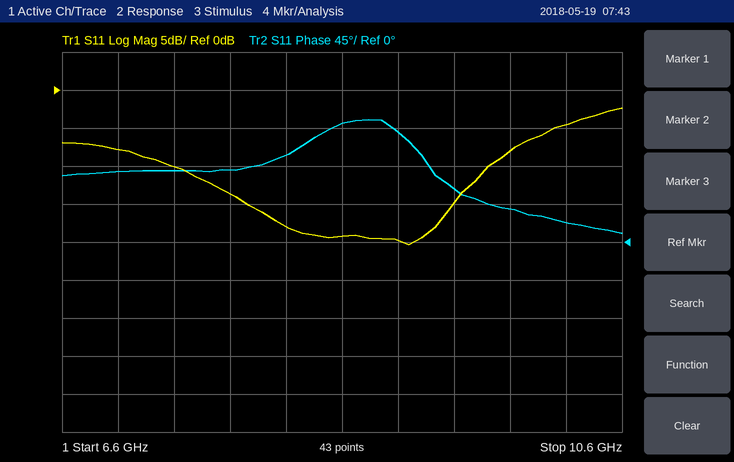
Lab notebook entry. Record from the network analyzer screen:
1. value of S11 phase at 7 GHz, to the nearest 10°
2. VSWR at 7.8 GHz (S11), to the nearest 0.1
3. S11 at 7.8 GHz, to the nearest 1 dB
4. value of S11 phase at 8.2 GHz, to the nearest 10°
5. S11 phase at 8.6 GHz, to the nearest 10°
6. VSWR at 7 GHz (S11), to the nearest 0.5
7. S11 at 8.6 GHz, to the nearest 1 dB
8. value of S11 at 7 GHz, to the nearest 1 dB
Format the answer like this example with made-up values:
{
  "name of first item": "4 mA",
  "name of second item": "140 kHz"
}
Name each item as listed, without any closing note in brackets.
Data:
{
  "value of S11 phase at 7 GHz, to the nearest 10°": "80°",
  "VSWR at 7.8 GHz (S11), to the nearest 0.1": "1.5",
  "S11 at 7.8 GHz, to the nearest 1 dB": "-14 dB",
  "value of S11 phase at 8.2 GHz, to the nearest 10°": "100°",
  "S11 phase at 8.6 GHz, to the nearest 10°": "140°",
  "VSWR at 7 GHz (S11), to the nearest 0.5": "2.5",
  "S11 at 8.6 GHz, to the nearest 1 dB": "-19 dB",
  "value of S11 at 7 GHz, to the nearest 1 dB": "-8 dB"
}
